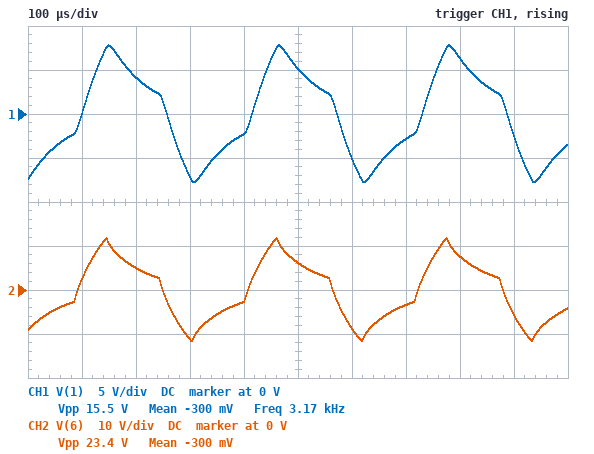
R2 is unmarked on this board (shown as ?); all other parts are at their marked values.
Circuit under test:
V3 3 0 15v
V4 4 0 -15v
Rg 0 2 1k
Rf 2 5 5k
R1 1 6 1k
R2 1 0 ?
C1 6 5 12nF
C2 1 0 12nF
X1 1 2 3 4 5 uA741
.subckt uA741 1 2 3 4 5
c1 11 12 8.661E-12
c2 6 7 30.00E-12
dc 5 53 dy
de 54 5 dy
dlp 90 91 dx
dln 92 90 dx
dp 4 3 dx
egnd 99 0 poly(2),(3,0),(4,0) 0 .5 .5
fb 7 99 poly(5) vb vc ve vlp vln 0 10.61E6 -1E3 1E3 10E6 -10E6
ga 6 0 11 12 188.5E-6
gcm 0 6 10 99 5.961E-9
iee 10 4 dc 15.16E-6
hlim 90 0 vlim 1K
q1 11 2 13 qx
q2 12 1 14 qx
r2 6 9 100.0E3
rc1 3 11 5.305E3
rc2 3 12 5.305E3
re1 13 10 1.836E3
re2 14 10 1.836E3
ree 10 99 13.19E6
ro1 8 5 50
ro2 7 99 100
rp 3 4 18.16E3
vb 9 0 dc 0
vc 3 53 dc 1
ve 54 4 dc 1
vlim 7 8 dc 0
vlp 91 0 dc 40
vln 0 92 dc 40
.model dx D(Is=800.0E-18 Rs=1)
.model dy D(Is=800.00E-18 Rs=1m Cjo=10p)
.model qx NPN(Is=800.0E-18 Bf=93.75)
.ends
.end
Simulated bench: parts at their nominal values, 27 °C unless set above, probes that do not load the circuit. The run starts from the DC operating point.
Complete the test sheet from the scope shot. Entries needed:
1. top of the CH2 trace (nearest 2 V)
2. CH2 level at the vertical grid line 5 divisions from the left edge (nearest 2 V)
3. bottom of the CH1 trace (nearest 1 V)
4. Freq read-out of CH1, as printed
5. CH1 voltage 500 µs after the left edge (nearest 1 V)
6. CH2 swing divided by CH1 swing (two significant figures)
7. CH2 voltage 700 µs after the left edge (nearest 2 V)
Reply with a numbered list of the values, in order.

1. 12 V
2. 6 V
3. -8 V
4. 3.17 kHz
5. 5 V
6. 1.5
7. -4 V
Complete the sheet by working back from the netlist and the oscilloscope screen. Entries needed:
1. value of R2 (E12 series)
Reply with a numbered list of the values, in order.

1. 2.7 kΩ
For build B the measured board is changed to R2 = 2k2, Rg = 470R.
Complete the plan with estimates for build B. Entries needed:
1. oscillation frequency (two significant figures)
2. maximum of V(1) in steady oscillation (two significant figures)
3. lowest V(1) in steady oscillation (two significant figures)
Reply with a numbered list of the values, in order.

1. 2.8 kHz
2. 7.6 V
3. -7.5 V
